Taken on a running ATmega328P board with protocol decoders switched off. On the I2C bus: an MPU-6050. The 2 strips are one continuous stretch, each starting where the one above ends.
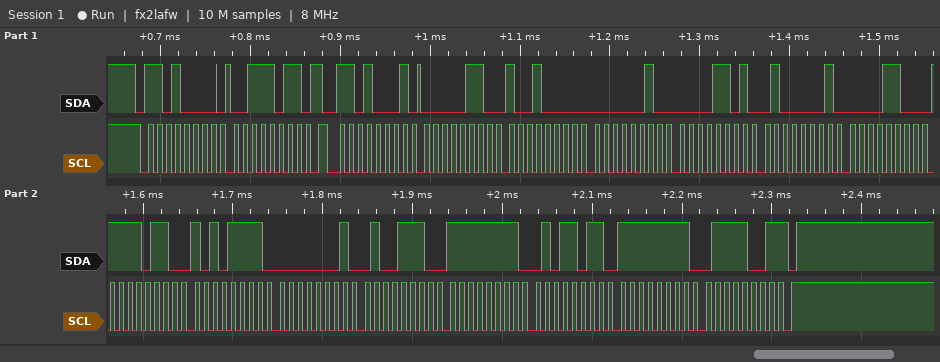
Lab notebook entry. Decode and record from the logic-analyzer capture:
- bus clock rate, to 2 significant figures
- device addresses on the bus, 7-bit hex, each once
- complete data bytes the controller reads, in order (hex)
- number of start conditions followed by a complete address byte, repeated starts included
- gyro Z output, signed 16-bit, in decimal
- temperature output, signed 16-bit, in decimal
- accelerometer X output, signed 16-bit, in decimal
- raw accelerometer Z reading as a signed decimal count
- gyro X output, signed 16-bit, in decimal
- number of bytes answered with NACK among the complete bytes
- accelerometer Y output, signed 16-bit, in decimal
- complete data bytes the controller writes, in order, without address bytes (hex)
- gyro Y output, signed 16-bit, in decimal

100 kHz
0x68
06 90 02 0D 41 0C F6 AF 01 4E FF 5B FF 79
2
-135
-2385
1680
16652
334
1
525
3B
-165
